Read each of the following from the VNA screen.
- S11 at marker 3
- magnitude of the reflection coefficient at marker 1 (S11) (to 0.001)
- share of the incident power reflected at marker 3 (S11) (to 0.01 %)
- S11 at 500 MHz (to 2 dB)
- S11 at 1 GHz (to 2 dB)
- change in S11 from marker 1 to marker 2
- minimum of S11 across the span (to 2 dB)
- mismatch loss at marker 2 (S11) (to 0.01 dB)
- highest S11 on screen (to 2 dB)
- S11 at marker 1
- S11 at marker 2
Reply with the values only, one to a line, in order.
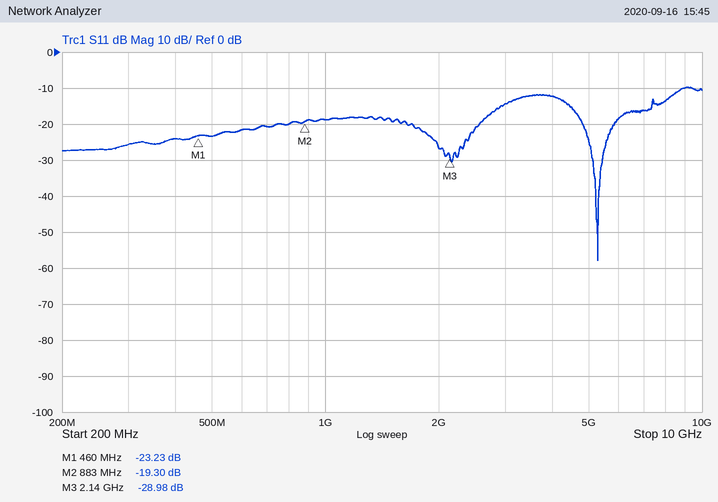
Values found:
-28.98 dB
0.069
0.13 %
-24 dB
-18 dB
3.93 dB
-58 dB
0.05 dB
-10 dB
-23.23 dB
-19.30 dB
